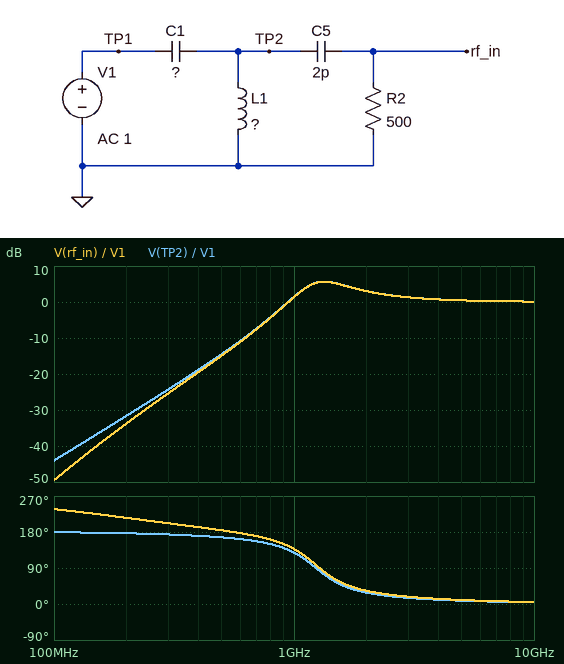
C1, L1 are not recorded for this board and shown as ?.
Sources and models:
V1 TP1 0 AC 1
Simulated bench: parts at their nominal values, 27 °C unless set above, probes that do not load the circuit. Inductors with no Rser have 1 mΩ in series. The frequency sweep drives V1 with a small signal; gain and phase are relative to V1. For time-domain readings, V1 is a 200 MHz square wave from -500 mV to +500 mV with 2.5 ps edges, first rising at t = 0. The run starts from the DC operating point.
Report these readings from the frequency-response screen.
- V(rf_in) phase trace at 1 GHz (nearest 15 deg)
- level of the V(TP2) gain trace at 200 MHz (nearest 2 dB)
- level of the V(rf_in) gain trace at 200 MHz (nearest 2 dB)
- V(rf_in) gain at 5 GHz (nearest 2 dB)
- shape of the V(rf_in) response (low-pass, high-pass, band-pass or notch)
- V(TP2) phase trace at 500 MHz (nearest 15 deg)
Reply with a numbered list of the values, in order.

1. 135 deg
2. -32 dB
3. -34 dB
4. 0 dB
5. high-pass
6. 165 deg
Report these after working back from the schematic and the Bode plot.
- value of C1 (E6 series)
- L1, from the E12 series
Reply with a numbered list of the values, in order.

1. 470 fF
2. 33 nH
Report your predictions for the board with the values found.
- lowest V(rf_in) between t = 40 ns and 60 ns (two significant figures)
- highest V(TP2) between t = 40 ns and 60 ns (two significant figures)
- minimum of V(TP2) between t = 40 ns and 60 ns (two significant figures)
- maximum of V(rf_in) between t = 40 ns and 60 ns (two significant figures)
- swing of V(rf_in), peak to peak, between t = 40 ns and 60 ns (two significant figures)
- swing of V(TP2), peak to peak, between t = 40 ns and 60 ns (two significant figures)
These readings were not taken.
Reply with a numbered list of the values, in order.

1. -990 mV
2. 990 mV
3. -990 mV
4. 990 mV
5. 2.0 V
6. 2.0 V
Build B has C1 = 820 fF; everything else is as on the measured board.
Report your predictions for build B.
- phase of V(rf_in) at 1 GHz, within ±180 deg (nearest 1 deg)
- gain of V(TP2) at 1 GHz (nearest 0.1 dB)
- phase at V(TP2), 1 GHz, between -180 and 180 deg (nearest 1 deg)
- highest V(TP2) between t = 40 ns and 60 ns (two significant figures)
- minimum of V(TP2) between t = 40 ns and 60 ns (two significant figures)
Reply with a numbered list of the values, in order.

1. 81 deg
2. 8.0 dB
3. 72 deg
4. 1.0 V
5. -1.0 V
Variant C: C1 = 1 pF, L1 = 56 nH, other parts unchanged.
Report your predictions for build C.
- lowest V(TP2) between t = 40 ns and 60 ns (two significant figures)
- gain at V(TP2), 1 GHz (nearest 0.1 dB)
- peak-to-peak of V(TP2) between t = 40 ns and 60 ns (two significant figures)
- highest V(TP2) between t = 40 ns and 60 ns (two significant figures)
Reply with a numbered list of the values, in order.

1. -1.1 V
2. 3.4 dB
3. 2.2 V
4. 1.1 V
